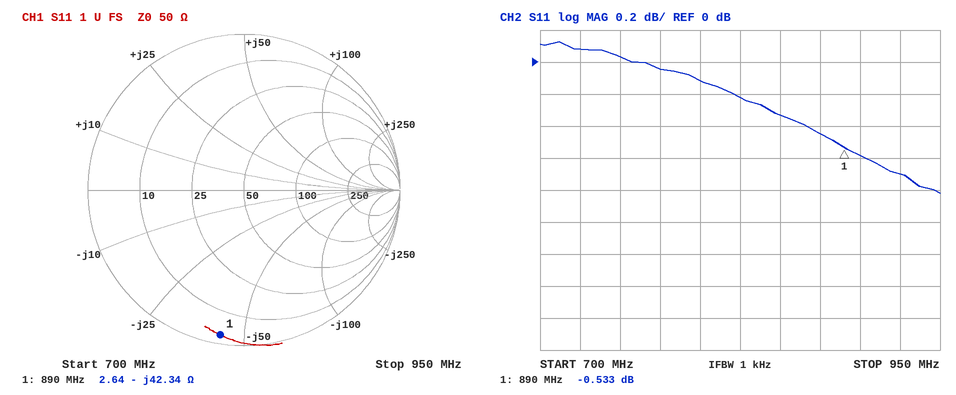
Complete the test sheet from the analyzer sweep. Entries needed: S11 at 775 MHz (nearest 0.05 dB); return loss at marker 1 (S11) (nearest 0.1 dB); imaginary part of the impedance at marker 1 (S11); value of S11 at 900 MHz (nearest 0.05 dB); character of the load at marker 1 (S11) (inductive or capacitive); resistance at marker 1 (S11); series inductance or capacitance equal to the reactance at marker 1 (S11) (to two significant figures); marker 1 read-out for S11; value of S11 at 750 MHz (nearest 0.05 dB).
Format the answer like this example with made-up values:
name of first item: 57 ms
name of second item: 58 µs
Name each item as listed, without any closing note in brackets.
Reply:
S11 at 775 MHz: -0.05 dB
return loss at marker 1 (S11): 0.5 dB
imaginary part of the impedance at marker 1: -42.34 Ω
value of S11 at 900 MHz: -0.60 dB
character of the load at marker 1 (S11): capacitive
resistance at marker 1: 2.64 Ω
series inductance or capacitance equal to the reactance at marker 1 (S11): 4.2 pF
marker 1 read-out for S11: -0.533 dB
value of S11 at 750 MHz: 0.05 dB
